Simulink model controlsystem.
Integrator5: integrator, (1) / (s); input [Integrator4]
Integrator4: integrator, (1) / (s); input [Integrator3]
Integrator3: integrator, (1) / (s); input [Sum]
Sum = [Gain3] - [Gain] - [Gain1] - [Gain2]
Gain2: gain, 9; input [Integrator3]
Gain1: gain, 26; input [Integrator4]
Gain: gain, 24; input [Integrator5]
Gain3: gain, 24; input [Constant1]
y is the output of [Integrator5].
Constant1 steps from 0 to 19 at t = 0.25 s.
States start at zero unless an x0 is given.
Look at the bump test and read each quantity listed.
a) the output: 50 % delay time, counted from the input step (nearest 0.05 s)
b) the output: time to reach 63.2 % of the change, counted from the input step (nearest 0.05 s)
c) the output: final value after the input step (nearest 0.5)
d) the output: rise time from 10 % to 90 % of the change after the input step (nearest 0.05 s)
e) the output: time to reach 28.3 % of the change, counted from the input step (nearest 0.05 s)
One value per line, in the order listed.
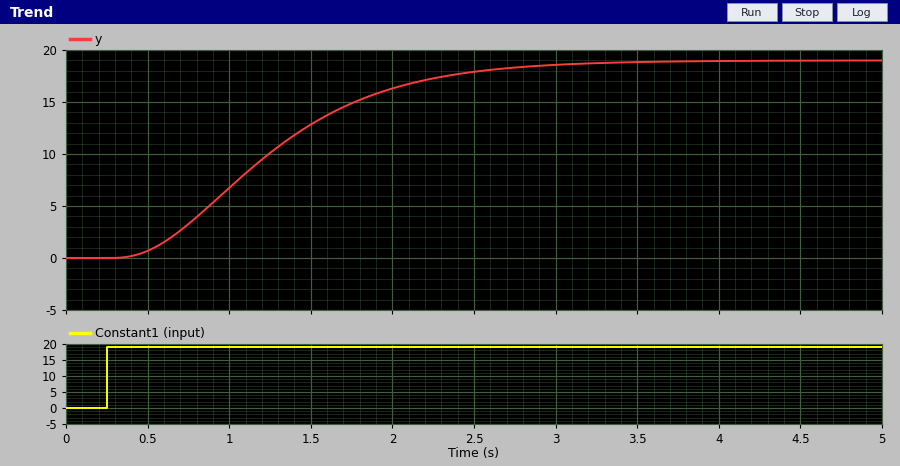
0.95 s
1.15 s
19.0
1.55 s
0.65 s
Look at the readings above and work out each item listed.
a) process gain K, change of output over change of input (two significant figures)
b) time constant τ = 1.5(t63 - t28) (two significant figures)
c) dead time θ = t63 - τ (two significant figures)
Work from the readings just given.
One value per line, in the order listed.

1.0
0.75 s
0.40 s
